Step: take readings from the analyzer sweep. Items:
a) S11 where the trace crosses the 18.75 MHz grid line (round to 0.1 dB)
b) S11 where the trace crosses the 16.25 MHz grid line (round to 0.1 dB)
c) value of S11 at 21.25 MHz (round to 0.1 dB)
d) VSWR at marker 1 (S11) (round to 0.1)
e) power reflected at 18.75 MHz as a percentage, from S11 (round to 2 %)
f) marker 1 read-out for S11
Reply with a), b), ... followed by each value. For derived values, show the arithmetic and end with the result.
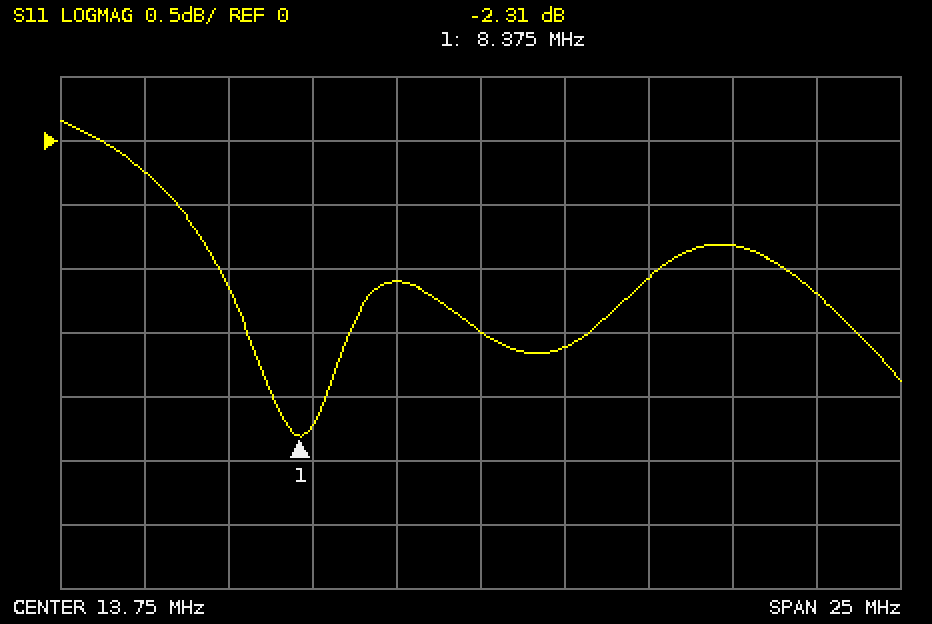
a) -1.1 dB
b) -1.6 dB
c) -0.8 dB
d) (1 + 0.7665)/(1 − 0.7665) ≈ 7.6
e) 10^(-1.1/10) ≈ 78 %
f) -2.31 dB
